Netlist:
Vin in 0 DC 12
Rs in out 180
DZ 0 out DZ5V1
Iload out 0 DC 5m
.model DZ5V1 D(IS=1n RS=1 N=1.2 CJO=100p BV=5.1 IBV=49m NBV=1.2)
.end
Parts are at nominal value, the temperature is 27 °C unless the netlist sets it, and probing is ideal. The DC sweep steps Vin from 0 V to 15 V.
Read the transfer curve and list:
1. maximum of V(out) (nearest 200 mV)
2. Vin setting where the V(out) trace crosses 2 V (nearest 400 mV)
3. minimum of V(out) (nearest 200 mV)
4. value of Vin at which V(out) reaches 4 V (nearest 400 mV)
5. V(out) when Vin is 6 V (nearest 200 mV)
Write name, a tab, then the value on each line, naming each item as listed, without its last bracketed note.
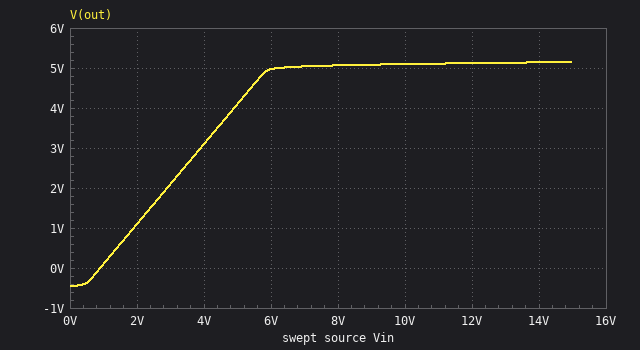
maximum of V(out)	5.2 V
Vin setting where the V(out) trace crosses 2 V	2.8 V
minimum of V(out)	-400 mV
value of Vin at which V(out) reaches 4 V	4.8 V
V(out) when Vin is 6 V	5.0 V
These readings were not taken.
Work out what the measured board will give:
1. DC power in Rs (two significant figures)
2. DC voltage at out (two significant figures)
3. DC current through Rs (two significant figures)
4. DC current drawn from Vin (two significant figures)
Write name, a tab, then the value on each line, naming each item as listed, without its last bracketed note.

DC power in Rs	260 mW
DC voltage at out	5.1 V
DC current through Rs	38 mA
DC current drawn from Vin	38 mA
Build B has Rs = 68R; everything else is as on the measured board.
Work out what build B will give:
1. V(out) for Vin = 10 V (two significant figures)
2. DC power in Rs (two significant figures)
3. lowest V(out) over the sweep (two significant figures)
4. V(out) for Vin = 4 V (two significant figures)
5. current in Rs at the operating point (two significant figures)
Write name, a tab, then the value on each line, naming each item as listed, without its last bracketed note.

V(out) for Vin = 10 V	5.2 V
DC power in Rs	680 mW
lowest V(out) over the sweep	-340 mV
V(out) for Vin = 4 V	3.7 V
current in Rs at the operating point	100 mA
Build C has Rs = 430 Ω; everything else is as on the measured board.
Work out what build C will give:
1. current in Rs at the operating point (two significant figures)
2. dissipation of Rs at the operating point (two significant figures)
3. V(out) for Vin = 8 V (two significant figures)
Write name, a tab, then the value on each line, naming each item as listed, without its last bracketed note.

current in Rs at the operating point	16 mA
dissipation of Rs at the operating point	110 mW
V(out) for Vin = 8 V	5.0 V
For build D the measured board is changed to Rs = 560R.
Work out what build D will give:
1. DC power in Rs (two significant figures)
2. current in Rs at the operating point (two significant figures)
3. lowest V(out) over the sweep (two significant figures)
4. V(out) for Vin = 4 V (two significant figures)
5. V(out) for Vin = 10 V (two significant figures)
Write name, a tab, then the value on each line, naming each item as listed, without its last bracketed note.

DC power in Rs	86 mW
current in Rs at the operating point	12 mA
lowest V(out) over the sweep	-480 mV
V(out) for Vin = 4 V	1.2 V
V(out) for Vin = 10 V	5.0 V
